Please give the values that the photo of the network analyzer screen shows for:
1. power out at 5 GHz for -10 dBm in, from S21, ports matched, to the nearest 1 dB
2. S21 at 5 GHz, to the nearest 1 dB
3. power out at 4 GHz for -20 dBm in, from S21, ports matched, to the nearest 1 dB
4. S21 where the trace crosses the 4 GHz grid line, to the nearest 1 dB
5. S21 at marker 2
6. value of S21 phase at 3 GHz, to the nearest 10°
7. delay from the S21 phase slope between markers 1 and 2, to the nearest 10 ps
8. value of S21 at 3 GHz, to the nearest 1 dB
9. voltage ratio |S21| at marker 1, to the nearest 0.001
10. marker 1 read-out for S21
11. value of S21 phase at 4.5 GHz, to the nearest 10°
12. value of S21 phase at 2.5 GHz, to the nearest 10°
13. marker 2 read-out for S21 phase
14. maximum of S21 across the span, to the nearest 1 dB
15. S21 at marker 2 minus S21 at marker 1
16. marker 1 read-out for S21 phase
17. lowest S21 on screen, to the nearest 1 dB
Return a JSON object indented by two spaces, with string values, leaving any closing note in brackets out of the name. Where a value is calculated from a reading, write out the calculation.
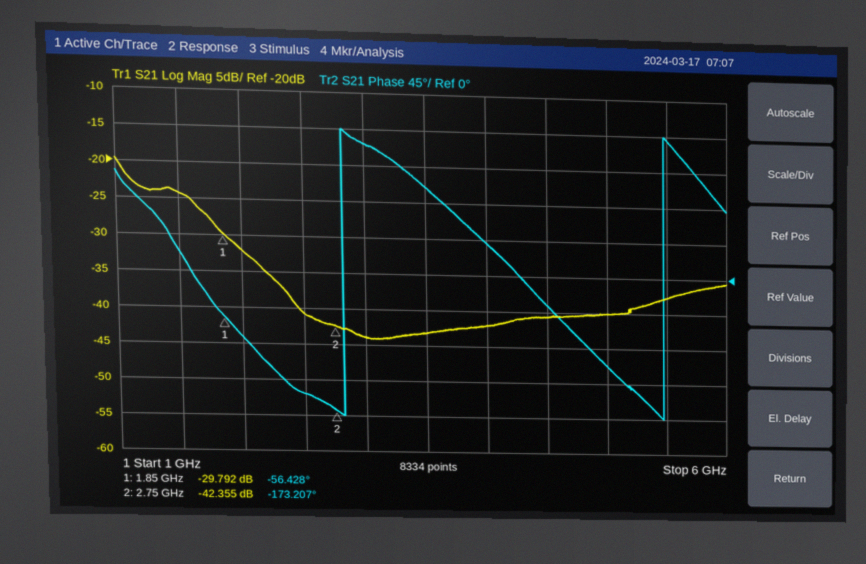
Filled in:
{
  "power out at 5 GHz for -10 dBm in, from S21, ports matched, to the nearest 1 dB": "-10 dBm + (-40 dB) = -50 dBm",
  "S21 at 5 GHz, to the nearest 1 dB": "-40 dB",
  "power out at 4 GHz for -20 dBm in, from S21, ports matched, to the nearest 1 dB": "-20 dBm + (-42 dB) = -62 dBm",
  "S21 where the trace crosses the 4 GHz grid line, to the nearest 1 dB": "-42 dB",
  "S21 at marker 2": "-42.355 dB",
  "value of S21 phase at 3 GHz, to the nearest 10°": "160°",
  "delay from the S21 phase slope between markers 1 and 2, to the nearest 10 ps": "−(-173.207° − (-56.428°))/(360° × 900 MHz) ≈ 360 ps",
  "value of S21 at 3 GHz, to the nearest 1 dB": "-44 dB",
  "voltage ratio |S21| at marker 1, to the nearest 0.001": "10^(-29.792/20) ≈ 0.032",
  "marker 1 read-out for S21": "-29.792 dB",
  "value of S21 phase at 4.5 GHz, to the nearest 10°": "-40°",
  "value of S21 phase at 2.5 GHz, to the nearest 10°": "-150°",
  "marker 2 read-out for S21 phase": "-173.207°",
  "maximum of S21 across the span, to the nearest 1 dB": "-20 dB",
  "S21 at marker 2 minus S21 at marker 1": "-42.355 − (-29.792) = -12.563 dB",
  "marker 1 read-out for S21 phase": "-56.428°",
  "lowest S21 on screen, to the nearest 1 dB": "-44 dB"
}
